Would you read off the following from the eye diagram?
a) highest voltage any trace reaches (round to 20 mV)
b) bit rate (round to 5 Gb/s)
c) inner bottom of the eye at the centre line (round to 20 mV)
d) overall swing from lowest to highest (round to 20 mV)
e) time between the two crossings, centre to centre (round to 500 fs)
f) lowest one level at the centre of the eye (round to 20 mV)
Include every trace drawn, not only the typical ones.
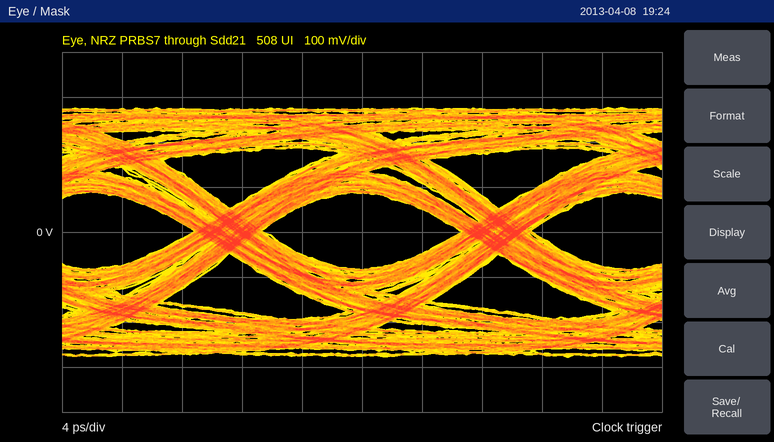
280 mV
55 Gb/s
-80 mV
560 mV
18.0 ps
80 mV
